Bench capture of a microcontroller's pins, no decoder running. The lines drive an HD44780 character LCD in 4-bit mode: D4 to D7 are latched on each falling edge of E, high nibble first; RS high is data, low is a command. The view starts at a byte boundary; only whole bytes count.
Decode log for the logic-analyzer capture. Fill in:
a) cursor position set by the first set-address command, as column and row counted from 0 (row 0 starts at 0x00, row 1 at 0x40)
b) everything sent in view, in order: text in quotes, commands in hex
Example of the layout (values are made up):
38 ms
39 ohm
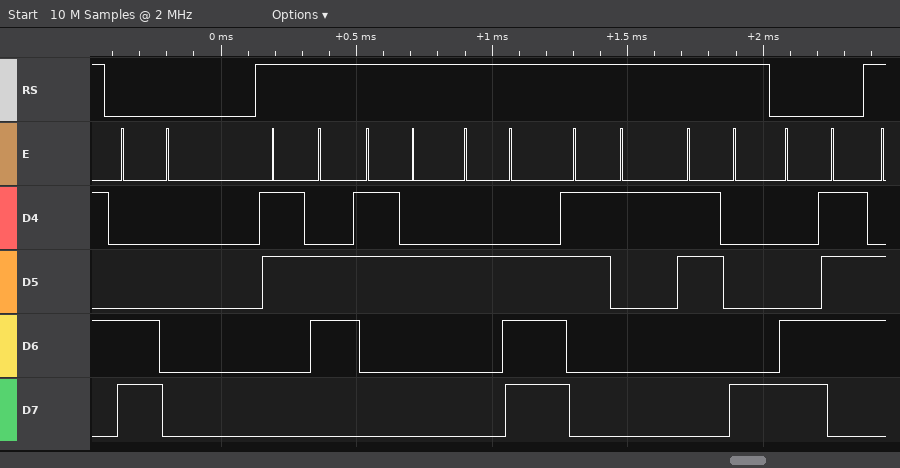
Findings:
column 0, row 1
0xC0 "62.18" 0xC7
